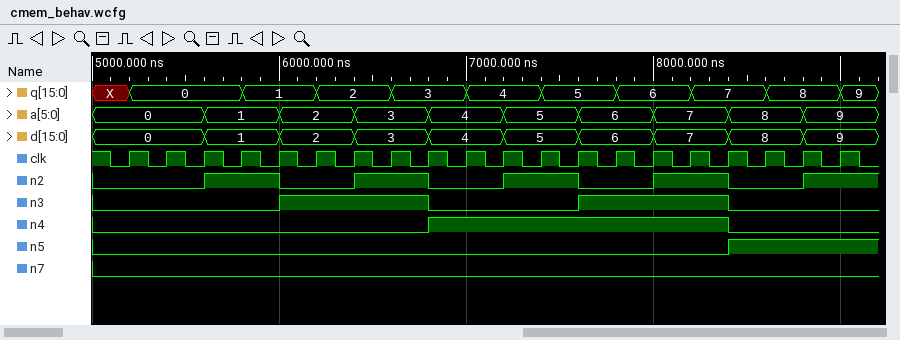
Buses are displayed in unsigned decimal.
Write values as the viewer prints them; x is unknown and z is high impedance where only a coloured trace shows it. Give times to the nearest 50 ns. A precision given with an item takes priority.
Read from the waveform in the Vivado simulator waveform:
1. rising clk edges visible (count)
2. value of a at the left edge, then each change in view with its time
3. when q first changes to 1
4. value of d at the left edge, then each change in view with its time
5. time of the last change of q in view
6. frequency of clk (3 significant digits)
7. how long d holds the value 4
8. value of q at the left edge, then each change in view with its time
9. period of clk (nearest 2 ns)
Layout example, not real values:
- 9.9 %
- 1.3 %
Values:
- 20
- 0, 1 at 5600 ns, 2 at 6000 ns, 3 at 6400 ns, 4 at 6800 ns, 5 at 7200 ns, 6 at 7600 ns, 7 at 8000 ns, 8 at 8400 ns, 9 at 8800 ns
- 5800 ns
- 0, 1 at 5600 ns, 2 at 6000 ns, 3 at 6400 ns, 4 at 6800 ns, 5 at 7200 ns, 6 at 7600 ns, 7 at 8000 ns, 8 at 8400 ns, 9 at 8800 ns
- 9000 ns
- 5.00 MHz
- 400 ns
- X, 0 at 5200 ns, 1 at 5800 ns, 2 at 6200 ns, 3 at 6600 ns, 4 at 7000 ns, 5 at 7400 ns, 6 at 7800 ns, 7 at 8200 ns, 8 at 8600 ns, 9 at 9000 ns
- 200 ns
